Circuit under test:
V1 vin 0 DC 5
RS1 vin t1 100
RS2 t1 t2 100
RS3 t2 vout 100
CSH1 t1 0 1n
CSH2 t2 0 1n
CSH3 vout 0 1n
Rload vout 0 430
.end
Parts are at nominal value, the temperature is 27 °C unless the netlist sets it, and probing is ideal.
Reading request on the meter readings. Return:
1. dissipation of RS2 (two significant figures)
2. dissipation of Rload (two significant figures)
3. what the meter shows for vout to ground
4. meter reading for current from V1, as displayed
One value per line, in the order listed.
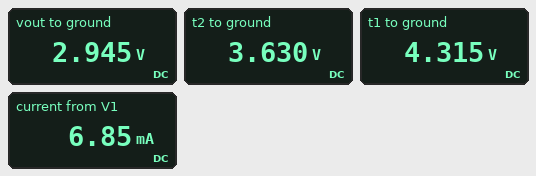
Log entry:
4.7 mW
20 mW
2.945 V
6.85 mA
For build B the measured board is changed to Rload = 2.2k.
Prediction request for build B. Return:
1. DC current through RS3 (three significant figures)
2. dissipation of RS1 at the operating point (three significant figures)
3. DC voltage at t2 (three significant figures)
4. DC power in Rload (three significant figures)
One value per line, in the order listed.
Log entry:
2.00 mA
400 µW
4.60 V
8.80 mW
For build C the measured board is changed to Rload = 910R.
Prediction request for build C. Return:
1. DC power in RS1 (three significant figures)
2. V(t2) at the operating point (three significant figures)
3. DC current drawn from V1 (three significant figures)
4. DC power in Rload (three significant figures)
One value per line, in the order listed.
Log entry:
1.71 mW
4.17 V
4.13 mA
15.5 mW
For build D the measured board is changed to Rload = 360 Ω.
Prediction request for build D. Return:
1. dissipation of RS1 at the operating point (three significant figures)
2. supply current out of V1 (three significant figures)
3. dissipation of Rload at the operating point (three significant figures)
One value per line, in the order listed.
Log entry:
5.74 mW
7.58 mA
20.7 mW
